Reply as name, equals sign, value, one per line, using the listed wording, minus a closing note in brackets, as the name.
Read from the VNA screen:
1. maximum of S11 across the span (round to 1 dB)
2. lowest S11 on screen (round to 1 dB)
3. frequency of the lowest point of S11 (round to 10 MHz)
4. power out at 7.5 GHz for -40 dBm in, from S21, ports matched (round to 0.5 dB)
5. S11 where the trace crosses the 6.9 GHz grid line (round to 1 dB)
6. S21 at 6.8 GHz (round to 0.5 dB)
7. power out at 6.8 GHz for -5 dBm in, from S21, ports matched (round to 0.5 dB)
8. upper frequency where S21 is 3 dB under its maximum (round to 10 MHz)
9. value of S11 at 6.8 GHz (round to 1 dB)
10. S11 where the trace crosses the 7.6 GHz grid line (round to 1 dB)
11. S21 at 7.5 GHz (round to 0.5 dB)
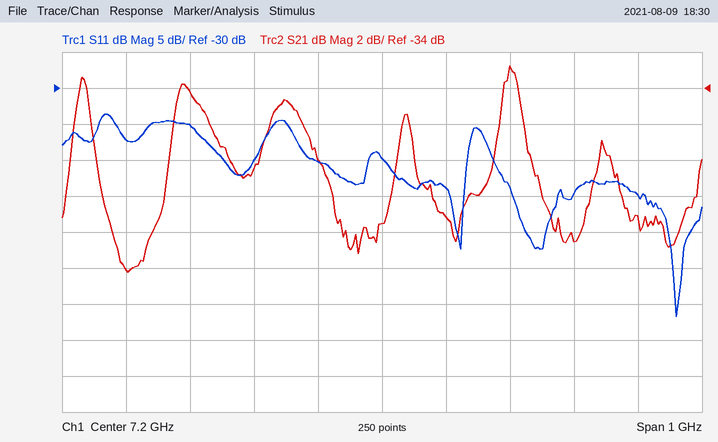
maximum of S11 across the span = -34 dB
lowest S11 on screen = -62 dB
frequency of the lowest point of S11 = 7.66 GHz
power out at 7.5 GHz for -40 dBm in, from S21, ports matched = -82.5 dBm
S11 where the trace crosses the 6.9 GHz grid line = -35 dB
S21 at 6.8 GHz = -44.0 dB
power out at 6.8 GHz for -5 dBm in, from S21, ports matched = -49.0 dBm
upper frequency where S21 is 3 dB under its maximum = 7.42 GHz
value of S11 at 6.8 GHz = -37 dB
S11 where the trace crosses the 7.6 GHz grid line = -45 dB
S21 at 7.5 GHz = -42.5 dB
